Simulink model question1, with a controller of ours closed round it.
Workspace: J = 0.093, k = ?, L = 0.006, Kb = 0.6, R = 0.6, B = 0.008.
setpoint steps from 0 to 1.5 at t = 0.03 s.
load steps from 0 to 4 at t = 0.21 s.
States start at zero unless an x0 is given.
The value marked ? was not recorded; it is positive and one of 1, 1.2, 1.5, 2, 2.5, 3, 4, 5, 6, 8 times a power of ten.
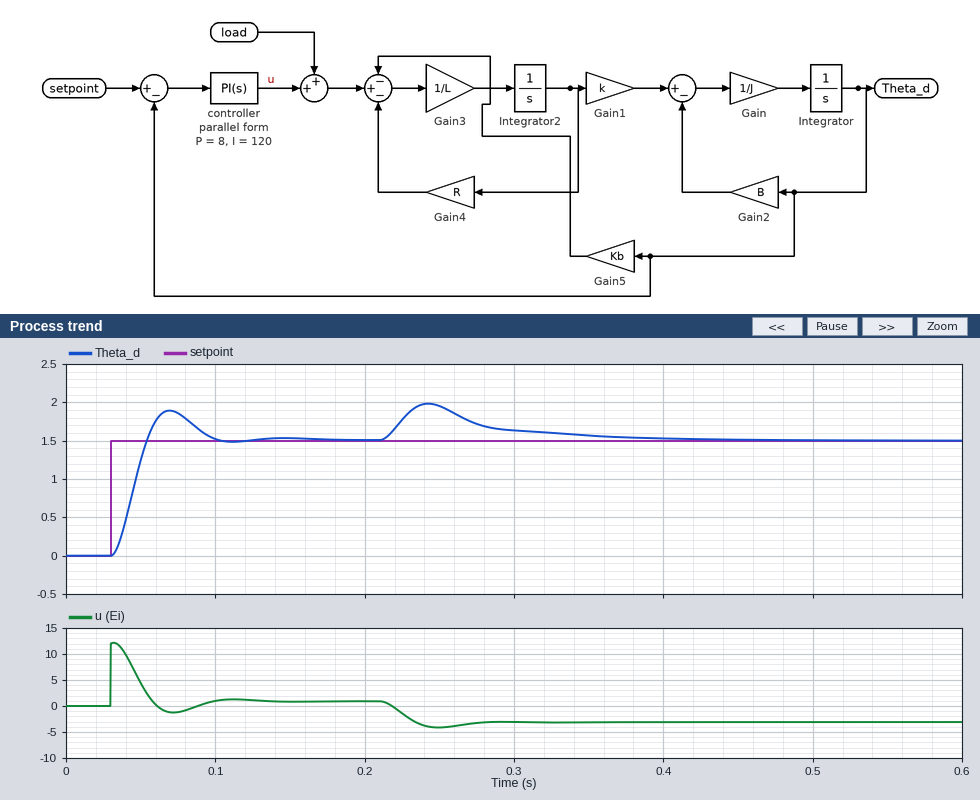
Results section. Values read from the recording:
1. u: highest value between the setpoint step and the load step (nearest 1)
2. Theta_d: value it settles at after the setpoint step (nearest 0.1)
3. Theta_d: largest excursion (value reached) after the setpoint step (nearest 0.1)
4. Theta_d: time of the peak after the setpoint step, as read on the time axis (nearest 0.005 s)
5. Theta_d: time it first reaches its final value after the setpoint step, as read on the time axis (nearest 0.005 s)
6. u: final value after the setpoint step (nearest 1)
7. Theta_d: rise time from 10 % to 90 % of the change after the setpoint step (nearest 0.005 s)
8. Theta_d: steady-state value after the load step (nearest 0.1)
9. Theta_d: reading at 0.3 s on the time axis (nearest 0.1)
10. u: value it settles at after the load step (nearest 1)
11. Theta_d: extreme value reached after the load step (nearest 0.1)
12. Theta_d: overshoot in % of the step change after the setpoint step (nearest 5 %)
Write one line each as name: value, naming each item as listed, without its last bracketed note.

u: highest value between the setpoint step and the load step: 12
Theta_d: value it settles at after the setpoint step: 1.5
Theta_d: largest excursion (value reached) after the setpoint step: 1.9
Theta_d: time of the peak after the setpoint step, as read on the time axis: 0.070 s
Theta_d: time it first reaches its final value after the setpoint step, as read on the time axis: 0.055 s
u: final value after the setpoint step: 1
Theta_d: rise time from 10 % to 90 % of the change after the setpoint step: 0.015 s
Theta_d: steady-state value after the load step: 1.5
Theta_d: reading at 0.3 s on the time axis: 1.6
u: value it settles at after the load step: -3
Theta_d: extreme value reached after the load step: 2.0
Theta_d: overshoot in % of the step change after the setpoint step: 25 %
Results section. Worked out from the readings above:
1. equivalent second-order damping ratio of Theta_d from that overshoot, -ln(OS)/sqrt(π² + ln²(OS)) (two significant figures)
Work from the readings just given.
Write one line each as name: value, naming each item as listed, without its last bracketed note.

equivalent second-order damping ratio of Theta_d from that overshoot, -ln(OS)/sqrt(π² + ln²(OS)): 0.40
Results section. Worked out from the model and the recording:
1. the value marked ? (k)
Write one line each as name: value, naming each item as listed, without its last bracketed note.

the value marked ?: 0.6
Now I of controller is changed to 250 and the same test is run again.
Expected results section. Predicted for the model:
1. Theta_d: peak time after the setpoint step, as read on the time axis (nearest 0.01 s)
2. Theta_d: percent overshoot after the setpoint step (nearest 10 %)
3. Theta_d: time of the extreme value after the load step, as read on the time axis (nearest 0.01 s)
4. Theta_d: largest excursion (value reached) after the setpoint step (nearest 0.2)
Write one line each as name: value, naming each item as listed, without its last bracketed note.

Theta_d: peak time after the setpoint step, as read on the time axis: 0.07 s
Theta_d: percent overshoot after the setpoint step: 40 %
Theta_d: time of the extreme value after the load step, as read on the time axis: 0.24 s
Theta_d: largest excursion (value reached) after the setpoint step: 2.2
